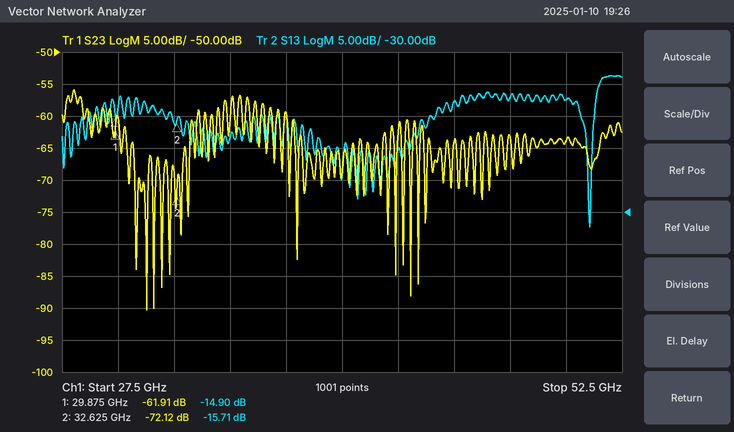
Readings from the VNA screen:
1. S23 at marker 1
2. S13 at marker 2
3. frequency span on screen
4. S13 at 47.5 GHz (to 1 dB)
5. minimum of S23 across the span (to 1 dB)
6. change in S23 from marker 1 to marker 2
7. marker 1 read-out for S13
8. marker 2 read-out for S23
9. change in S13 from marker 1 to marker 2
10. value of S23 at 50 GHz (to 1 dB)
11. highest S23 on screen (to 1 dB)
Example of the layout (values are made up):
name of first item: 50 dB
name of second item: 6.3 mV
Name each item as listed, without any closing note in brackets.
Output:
S23 at marker 1: -61.91 dB
S13 at marker 2: -15.71 dB
frequency span on screen: 25 GHz
S13 at 47.5 GHz: -12 dB
minimum of S23 across the span: -90 dB
change in S23 from marker 1 to marker 2: -10.21 dB
marker 1 read-out for S13: -14.90 dB
marker 2 read-out for S23: -72.12 dB
change in S13 from marker 1 to marker 2: -0.81 dB
value of S23 at 50 GHz: -64 dB
highest S23 on screen: -56 dB
